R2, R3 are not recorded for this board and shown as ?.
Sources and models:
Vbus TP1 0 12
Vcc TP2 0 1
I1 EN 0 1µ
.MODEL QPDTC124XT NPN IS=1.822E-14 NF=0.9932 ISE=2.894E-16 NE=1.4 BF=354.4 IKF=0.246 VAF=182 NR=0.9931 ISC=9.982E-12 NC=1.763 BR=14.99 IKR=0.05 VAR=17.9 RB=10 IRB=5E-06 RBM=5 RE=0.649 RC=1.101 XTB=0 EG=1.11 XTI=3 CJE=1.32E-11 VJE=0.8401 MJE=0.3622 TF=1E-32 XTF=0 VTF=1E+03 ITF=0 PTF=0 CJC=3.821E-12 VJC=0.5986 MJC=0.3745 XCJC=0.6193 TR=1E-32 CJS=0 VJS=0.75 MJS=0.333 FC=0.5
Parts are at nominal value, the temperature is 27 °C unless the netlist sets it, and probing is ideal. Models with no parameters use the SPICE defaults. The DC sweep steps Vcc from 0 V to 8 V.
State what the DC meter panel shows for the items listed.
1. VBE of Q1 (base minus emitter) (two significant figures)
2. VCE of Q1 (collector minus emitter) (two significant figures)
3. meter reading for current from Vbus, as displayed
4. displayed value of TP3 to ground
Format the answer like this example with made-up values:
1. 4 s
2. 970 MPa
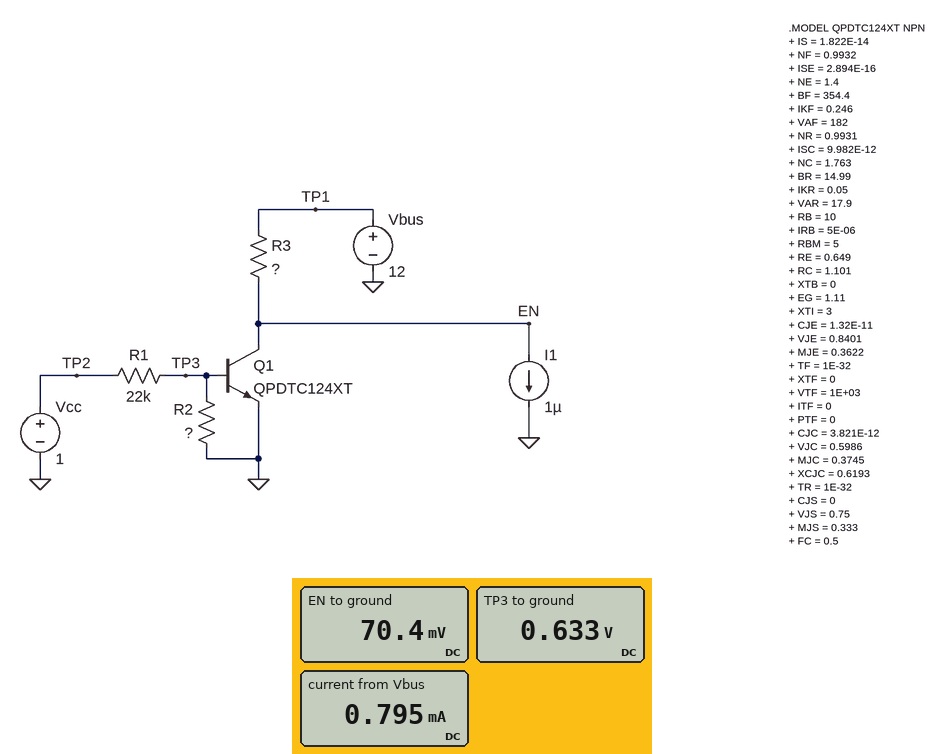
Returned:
1. 630 mV
2. 70 mV
3. 0.795 mA
4. 0.633 V
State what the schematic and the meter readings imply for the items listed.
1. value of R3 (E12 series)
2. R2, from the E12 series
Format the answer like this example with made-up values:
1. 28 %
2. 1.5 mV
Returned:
1. 15 kΩ
2. 82 kΩ
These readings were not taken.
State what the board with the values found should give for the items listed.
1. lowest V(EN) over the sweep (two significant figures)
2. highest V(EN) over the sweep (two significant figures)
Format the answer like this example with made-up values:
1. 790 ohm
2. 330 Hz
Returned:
1. 8.4 mV
2. 12 V
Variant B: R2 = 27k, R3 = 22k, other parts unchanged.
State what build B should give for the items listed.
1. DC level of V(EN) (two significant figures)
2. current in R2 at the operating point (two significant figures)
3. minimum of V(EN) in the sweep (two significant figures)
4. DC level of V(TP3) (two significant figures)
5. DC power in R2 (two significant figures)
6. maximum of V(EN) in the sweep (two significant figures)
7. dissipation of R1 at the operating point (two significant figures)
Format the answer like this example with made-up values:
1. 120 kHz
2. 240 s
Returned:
1. 11 V
2. 20 µA
3. 6.7 mV
4. 550 mV
5. 11 µW
6. 12 V
7. 9.2 µW
